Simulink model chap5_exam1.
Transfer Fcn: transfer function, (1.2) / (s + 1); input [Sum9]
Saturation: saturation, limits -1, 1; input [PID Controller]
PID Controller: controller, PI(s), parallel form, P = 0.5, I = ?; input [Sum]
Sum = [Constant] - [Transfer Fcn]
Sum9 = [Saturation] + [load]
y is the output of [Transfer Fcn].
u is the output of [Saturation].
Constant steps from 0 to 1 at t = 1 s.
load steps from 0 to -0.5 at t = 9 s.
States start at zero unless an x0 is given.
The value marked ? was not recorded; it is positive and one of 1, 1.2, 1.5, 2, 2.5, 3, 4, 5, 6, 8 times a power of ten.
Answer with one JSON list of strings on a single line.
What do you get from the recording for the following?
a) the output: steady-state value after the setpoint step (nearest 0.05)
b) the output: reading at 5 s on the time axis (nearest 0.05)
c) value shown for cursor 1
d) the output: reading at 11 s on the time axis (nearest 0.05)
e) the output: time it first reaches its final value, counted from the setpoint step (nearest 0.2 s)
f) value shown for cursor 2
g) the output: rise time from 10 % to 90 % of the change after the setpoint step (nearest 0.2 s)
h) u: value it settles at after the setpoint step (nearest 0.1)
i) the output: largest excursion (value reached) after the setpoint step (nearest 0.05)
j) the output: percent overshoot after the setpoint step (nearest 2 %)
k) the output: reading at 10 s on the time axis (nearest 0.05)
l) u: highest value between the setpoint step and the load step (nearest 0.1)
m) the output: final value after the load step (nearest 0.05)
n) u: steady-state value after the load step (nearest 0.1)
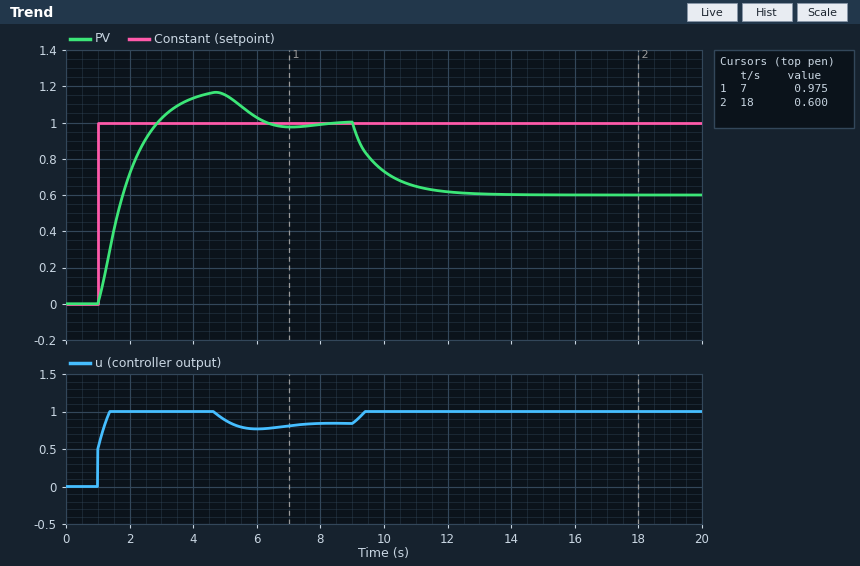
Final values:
["1.00", "1.15", "0.975", "0.65", "1.8 s", "0.600", "1.4 s", "0.8", "1.15", "16 %", "0.75", "1.0", "0.60", "1.0"]
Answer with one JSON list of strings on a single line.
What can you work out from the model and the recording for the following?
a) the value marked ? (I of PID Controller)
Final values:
["2"]
